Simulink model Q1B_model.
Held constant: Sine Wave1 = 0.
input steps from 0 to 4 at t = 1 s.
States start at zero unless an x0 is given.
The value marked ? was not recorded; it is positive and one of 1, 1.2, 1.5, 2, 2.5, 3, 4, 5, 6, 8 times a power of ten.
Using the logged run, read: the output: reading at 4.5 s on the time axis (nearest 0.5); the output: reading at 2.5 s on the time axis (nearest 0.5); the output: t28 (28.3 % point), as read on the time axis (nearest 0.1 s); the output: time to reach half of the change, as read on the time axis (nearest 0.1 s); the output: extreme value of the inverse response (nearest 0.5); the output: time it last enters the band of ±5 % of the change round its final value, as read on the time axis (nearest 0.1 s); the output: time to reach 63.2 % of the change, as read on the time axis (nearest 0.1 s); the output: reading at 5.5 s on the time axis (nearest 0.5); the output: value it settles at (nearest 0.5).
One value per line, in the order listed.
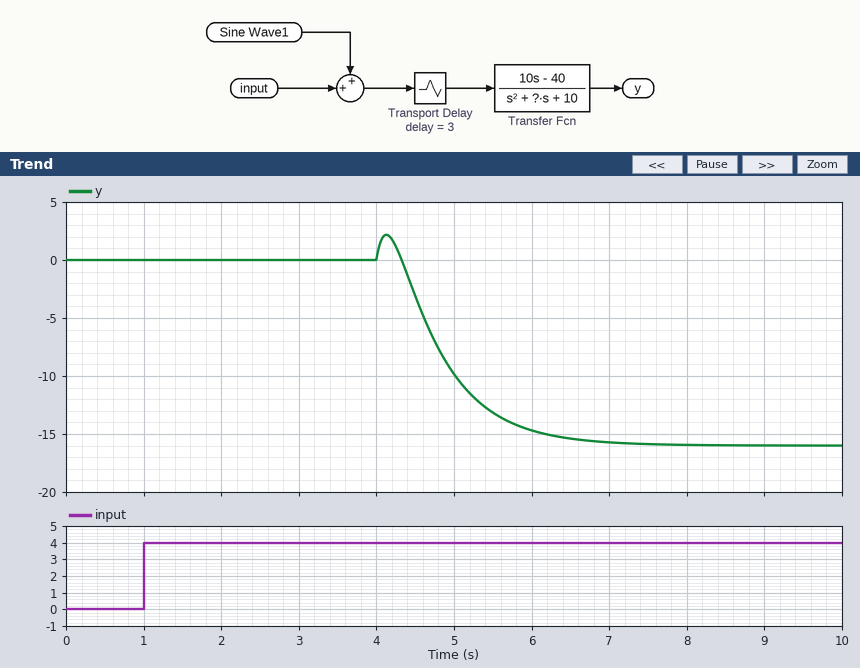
-3.0
0.0
4.6 s
4.8 s
2.0
6.3 s
5.0 s
-13.0
-16.0
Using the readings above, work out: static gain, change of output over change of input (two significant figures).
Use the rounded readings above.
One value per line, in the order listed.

-4.0
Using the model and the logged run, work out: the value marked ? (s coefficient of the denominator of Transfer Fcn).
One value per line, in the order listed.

8
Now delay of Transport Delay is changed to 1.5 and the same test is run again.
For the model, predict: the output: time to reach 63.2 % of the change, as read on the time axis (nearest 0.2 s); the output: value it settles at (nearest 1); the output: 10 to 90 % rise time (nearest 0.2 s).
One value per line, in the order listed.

3.6 s
-16
1.4 s
